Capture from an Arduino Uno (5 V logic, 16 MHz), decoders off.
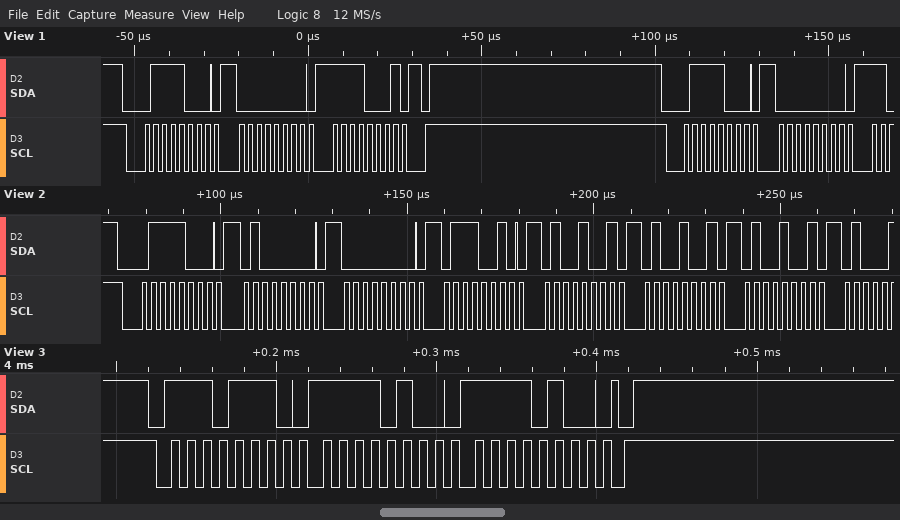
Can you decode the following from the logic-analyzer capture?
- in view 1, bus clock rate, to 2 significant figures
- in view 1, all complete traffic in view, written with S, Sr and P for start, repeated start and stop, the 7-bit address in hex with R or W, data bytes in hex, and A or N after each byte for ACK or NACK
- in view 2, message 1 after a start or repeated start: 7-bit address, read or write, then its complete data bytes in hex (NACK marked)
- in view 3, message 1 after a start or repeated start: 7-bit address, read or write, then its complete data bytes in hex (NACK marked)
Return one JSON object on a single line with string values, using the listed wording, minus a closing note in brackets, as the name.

{"in view 1, bus clock rate, to 2 significant figures": "400 kHz", "in view 1, all complete traffic in view, written with S, Sr and P for start, repeated start and stop, the 7-bit address in hex with R or W, data bytes in hex, and A or N after each byte for ACK or NACK": "S 3CW A 00 A F1 A P S 3CW A 00 A", "in view 2, message 1 after a start or repeated start: 7-bit address, read or write, then its complete data bytes in hex": "0x3C write: 40 00 72 49 49 49", "in view 3, message 1 after a start or repeated start: 7-bit address, read or write, then its complete data bytes in hex": "0x77 write: F4 F4"}
